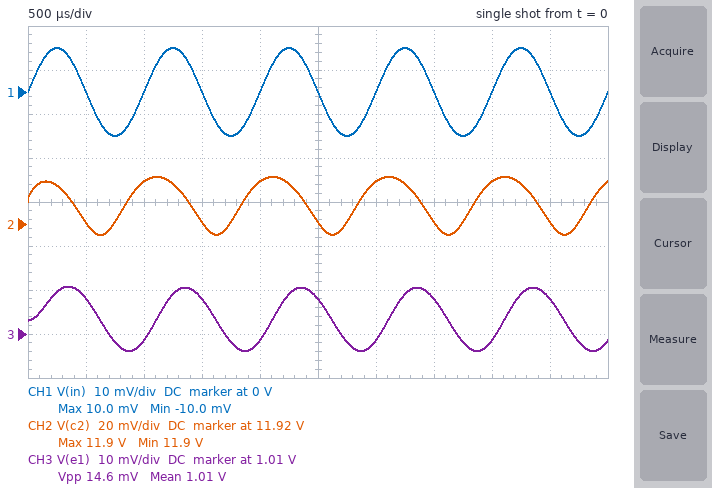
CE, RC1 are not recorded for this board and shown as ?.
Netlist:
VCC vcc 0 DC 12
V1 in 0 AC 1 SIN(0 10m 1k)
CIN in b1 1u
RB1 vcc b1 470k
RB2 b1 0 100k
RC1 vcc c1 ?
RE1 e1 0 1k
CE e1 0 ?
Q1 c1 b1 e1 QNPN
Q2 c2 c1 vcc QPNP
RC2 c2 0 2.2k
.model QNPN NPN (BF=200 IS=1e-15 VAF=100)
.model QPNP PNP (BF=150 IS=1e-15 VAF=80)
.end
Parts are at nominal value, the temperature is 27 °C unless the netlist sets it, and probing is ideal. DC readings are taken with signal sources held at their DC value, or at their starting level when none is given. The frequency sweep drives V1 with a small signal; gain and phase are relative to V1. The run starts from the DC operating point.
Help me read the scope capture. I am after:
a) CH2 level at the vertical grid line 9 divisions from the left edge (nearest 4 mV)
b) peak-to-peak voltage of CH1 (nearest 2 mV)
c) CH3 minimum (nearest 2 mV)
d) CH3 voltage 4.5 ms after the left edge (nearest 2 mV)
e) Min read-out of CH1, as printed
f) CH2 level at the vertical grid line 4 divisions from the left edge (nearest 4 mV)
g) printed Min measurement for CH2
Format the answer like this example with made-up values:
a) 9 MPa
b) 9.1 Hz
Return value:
a) 11.920 V
b) 20 mV
c) 1.006 V
d) 1.018 V
e) -10.0 mV
f) 11.940 V
g) 11.9 V
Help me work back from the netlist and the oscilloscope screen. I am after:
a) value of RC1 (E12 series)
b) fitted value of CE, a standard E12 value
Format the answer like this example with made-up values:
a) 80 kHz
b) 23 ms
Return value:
a) 1.5 kΩ
b) 5.6 µF
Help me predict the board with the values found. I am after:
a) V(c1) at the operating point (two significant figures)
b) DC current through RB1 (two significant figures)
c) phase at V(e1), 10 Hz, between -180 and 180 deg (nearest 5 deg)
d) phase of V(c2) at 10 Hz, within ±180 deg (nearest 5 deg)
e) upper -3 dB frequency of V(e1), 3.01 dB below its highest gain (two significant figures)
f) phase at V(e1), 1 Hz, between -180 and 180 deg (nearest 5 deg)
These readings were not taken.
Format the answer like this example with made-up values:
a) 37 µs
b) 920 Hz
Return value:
a) 11 V
b) 22 µA
c) 15 deg
d) 35 deg
e) 1.2 kHz
f) 70 deg
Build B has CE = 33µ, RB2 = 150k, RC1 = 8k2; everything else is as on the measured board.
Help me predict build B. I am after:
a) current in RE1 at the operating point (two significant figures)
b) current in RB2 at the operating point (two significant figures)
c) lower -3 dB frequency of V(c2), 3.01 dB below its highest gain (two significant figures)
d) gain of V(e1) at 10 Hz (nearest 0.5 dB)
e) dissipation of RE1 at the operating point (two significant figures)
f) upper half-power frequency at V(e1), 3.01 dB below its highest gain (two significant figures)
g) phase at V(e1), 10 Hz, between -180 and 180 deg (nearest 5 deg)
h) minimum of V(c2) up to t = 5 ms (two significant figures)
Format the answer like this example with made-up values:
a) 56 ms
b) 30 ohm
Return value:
a) 1.4 mA
b) 14 µA
c) 310 Hz
d) -1.5 dB
e) 2.1 mW
f) 320 Hz
g) 10 deg
h) 12 V
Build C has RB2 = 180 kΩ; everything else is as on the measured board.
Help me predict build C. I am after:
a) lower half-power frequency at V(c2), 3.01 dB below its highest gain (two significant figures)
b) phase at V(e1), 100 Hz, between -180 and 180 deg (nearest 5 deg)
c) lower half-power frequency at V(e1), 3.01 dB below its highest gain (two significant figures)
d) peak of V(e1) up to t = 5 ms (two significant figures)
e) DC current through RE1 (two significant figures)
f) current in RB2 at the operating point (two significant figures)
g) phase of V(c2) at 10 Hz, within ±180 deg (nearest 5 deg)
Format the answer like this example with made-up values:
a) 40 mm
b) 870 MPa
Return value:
a) 1.9 kHz
b) 0 deg
c) 1.9 Hz
d) 1.6 V
e) 1.6 mA
f) 13 µA
g) 30 deg
